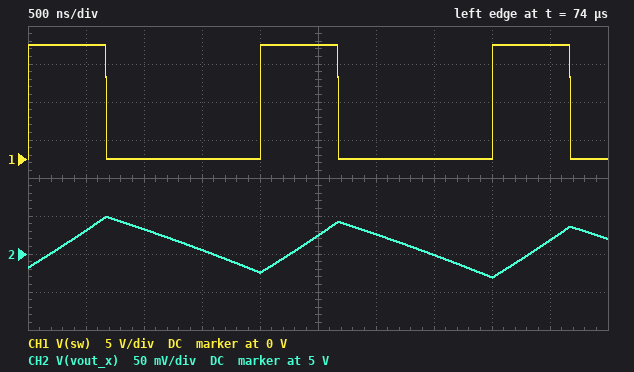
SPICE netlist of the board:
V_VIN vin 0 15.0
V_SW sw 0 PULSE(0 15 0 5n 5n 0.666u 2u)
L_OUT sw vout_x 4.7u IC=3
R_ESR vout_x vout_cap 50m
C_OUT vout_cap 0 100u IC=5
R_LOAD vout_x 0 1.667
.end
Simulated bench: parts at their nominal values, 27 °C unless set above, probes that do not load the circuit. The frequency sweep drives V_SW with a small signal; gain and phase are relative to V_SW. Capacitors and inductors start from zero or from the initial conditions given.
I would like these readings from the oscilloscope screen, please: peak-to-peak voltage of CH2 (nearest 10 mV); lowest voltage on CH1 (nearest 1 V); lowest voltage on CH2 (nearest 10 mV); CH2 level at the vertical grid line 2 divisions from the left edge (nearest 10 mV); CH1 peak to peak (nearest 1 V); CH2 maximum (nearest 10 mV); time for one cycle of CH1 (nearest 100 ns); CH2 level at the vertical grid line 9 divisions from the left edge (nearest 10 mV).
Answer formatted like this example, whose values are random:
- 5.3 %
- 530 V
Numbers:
- 80 mV
- 0 V
- 4.97 V
- 5.03 V
- 15 V
- 5.05 V
- 2.0 µs
- 5.02 V
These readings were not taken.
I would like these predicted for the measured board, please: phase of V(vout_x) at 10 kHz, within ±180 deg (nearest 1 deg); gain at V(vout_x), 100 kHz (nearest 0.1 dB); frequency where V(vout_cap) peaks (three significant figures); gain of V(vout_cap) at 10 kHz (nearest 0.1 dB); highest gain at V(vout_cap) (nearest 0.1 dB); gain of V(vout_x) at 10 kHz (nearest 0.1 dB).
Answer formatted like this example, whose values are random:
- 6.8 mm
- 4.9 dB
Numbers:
- -134 deg
- -35.2 dB
- 7.00 kHz
- -0.3 dB
- 9.1 dB
- 0.1 dB
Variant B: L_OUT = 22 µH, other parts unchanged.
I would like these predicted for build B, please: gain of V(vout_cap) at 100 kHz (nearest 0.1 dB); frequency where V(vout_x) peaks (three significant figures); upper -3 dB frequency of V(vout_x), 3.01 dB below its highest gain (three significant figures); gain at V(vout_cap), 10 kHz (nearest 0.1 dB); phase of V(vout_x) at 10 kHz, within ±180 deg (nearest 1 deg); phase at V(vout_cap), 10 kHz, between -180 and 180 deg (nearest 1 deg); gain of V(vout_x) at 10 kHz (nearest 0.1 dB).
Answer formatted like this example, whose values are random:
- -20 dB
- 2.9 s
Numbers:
- -59.0 dB
- 3.22 kHz
- 3.82 kHz
- -18.1 dB
- -154 deg
- -172 deg
- -17.7 dB
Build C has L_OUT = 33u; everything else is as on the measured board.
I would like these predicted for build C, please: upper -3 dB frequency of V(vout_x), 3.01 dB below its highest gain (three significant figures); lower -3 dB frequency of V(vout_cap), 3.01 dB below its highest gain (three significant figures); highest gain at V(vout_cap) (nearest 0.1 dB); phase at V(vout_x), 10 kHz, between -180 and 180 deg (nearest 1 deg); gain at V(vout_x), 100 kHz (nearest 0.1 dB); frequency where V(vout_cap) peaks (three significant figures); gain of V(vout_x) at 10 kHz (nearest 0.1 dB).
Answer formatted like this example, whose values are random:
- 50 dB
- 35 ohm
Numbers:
- 3.14 kHz
- 1.92 kHz
- 7.6 dB
- -155 deg
- -52.2 dB
- 2.60 kHz
- -21.5 dB
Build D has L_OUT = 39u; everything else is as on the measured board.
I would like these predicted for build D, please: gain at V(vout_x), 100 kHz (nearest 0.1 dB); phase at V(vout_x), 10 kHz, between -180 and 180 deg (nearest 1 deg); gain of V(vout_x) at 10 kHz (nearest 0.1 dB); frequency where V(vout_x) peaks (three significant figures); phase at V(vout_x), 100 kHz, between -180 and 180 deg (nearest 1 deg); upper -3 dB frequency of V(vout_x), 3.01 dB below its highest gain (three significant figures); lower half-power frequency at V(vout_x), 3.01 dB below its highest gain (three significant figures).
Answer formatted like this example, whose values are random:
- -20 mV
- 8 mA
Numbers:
- -53.6 dB
- -156 deg
- -23.1 dB
- 2.38 kHz
- -107 deg
- 2.90 kHz
- 1.71 kHz
